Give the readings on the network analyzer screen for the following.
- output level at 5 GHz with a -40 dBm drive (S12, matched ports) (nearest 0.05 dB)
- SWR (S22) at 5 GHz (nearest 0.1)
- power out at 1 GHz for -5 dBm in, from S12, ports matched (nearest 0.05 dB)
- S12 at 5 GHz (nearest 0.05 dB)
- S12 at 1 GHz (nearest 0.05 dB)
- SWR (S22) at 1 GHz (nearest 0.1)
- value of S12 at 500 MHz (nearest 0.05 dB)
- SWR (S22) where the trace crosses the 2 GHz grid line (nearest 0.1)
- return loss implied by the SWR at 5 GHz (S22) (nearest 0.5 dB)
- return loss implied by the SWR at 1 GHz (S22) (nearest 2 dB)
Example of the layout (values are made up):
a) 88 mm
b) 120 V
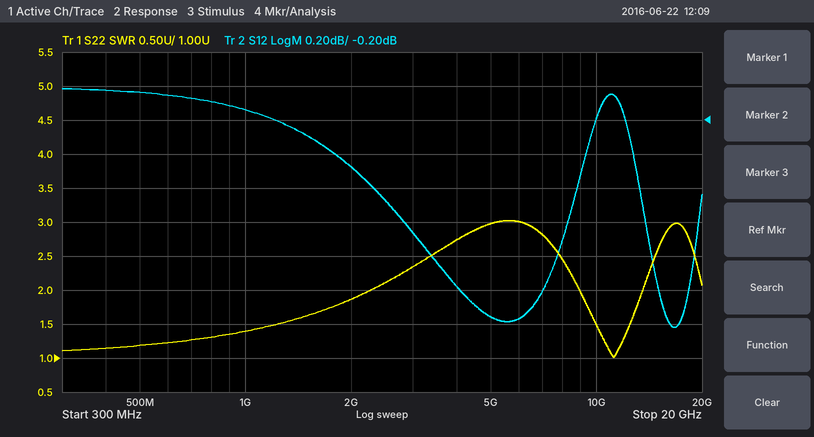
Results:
a) -41.35 dBm
b) 3.0
c) -5.15 dBm
d) -1.35 dB
e) -0.15 dB
f) 1.4
g) -0.05 dB
h) 1.9
i) 6.0 dB
j) 16 dB
